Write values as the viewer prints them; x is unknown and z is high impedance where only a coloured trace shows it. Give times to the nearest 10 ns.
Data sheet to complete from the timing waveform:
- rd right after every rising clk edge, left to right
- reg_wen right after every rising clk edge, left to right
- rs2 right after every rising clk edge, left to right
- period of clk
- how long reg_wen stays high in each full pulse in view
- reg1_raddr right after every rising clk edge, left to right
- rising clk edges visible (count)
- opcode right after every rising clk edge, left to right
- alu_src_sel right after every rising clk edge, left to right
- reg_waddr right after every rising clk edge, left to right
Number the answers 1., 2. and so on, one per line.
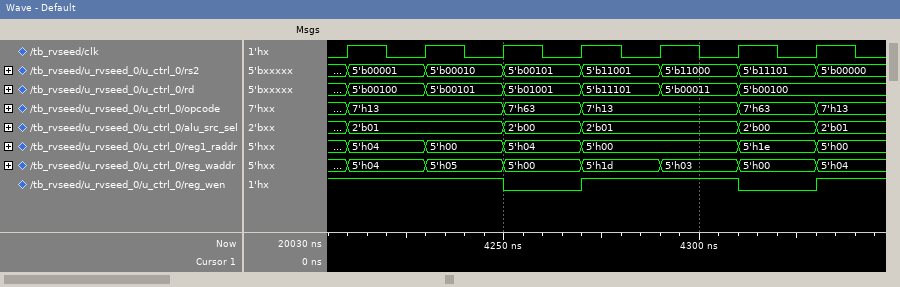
1. 5'b00100, 5'b00101, 5'b01001, 5'b11101, 5'b00011, 5'b00100, 5'b00100
2. 1 1 0 1 1 0 1
3. 5'b00001, 5'b00010, 5'b00101, 5'b11001, 5'b11000, 5'b11101, 5'b00000
4. 20 ns
5. 40 ns
6. 5'h04, 5'h00, 5'h04, 5'h00, 5'h00, 5'h1e, 5'h00
7. 7
8. 7'h13, 7'h13, 7'h63, 7'h13, 7'h13, 7'h63, 7'h13
9. 2'b01, 2'b01, 2'b00, 2'b01, 2'b01, 2'b00, 2'b01
10. 5'h04, 5'h05, 5'h00, 5'h1d, 5'h03, 5'h00, 5'h04
